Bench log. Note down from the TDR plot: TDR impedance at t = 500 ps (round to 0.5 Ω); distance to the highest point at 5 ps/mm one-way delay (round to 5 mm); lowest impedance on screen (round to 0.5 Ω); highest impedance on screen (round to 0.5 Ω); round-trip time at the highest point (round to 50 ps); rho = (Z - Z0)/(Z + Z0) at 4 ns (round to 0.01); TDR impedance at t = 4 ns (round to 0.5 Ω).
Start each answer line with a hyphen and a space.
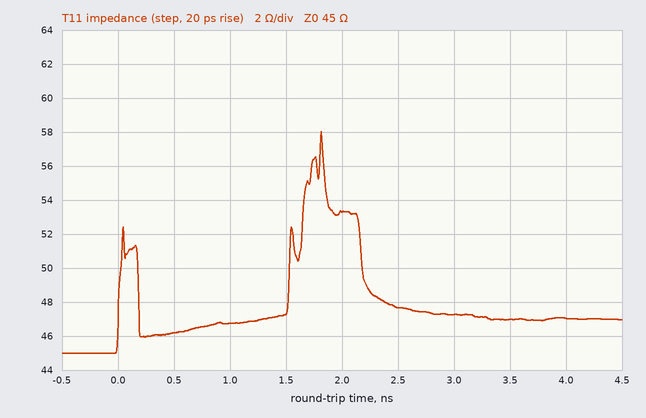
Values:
- 46.0 Ω
- 180 mm
- 45.0 Ω
- 58.0 Ω
- 1.80 ns
- +0.02
- 47.0 Ω
